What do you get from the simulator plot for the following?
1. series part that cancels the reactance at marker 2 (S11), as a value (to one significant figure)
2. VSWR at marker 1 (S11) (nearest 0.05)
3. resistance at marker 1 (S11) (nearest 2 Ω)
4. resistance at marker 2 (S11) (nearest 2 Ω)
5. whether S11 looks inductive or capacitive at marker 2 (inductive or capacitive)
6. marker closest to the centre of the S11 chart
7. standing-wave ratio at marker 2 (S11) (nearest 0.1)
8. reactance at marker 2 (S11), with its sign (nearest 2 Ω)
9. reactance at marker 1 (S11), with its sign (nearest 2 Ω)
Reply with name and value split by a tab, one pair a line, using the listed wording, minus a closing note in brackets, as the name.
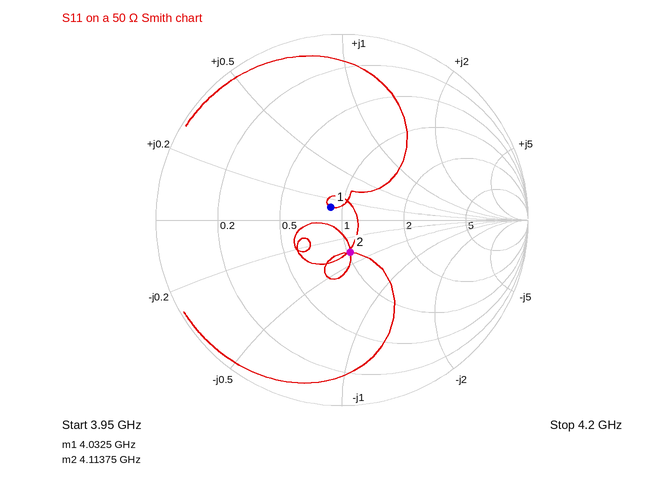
series part that cancels the reactance at marker 2 (S11), as a value	700 pH
VSWR at marker 1 (S11)	1.20
resistance at marker 1 (S11)	44 Ω
resistance at marker 2 (S11)	52 Ω
whether S11 looks inductive or capacitive at marker 2	capacitive
marker closest to the centre of the S11 chart	marker 1
standing-wave ratio at marker 2 (S11)	1.4
reactance at marker 2 (S11), with its sign	-18 Ω
reactance at marker 1 (S11), with its sign	+6 Ω
